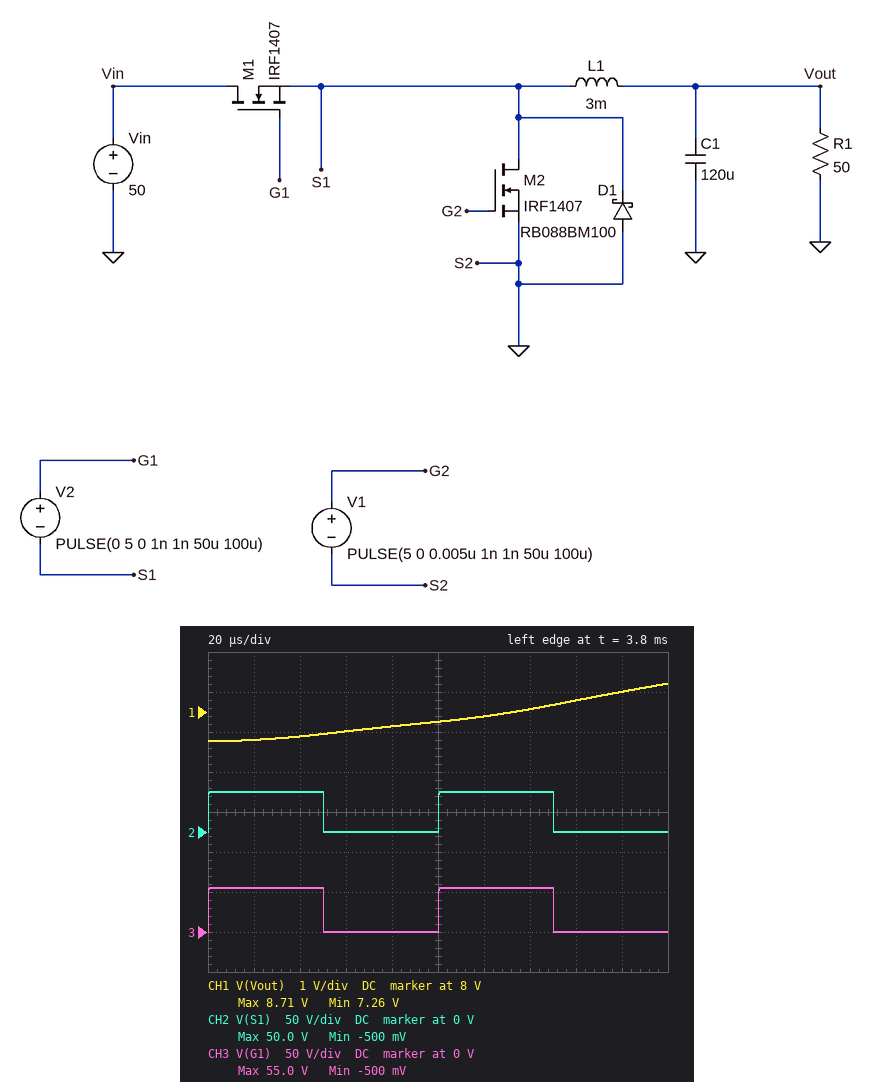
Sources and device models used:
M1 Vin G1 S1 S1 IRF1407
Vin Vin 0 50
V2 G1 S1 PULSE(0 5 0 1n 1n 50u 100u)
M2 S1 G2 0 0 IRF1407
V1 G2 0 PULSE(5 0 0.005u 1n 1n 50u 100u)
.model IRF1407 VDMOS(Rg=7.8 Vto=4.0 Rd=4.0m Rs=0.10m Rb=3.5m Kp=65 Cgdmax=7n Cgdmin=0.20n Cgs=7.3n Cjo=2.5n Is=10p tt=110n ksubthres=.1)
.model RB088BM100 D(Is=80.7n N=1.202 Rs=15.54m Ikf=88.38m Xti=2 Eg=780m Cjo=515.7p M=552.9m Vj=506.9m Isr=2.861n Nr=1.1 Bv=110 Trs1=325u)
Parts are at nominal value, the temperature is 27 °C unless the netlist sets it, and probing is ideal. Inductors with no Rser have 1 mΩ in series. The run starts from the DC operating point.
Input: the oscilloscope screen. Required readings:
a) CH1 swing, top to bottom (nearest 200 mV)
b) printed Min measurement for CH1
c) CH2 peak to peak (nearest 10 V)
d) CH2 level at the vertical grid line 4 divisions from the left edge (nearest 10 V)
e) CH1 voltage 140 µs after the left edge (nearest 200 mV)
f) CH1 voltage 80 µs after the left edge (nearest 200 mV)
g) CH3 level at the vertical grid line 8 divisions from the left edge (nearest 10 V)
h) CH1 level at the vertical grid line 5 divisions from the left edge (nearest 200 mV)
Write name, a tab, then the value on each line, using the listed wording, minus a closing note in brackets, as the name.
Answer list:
CH1 swing, top to bottom	1.4 V
printed Min measurement for CH1	7.26 V
CH2 peak to peak	50 V
CH2 level at the vertical grid line 4 divisions from the left edge	0 V
CH1 voltage 140 µs after the left edge	8.0 V
CH1 voltage 80 µs after the left edge	7.6 V
CH3 level at the vertical grid line 8 divisions from the left edge	0 V
CH1 level at the vertical grid line 5 divisions from the left edge	7.8 V
